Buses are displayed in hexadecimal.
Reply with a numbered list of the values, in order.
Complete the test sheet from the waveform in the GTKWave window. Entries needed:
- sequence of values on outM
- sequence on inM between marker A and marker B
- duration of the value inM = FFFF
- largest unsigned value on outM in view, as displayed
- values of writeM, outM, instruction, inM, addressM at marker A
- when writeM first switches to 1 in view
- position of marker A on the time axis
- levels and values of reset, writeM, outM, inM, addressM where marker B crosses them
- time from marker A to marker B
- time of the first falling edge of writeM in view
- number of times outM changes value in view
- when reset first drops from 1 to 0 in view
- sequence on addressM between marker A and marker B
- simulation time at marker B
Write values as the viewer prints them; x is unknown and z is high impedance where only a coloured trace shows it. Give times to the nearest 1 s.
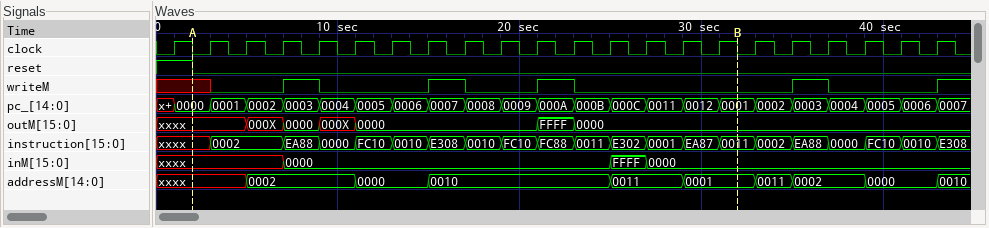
1. xxxx, 000X, 0000, 000X, 0000, FFFF, 0000
2. xxxx, 0000, FFFF, 0000
3. 2 s
4. FFFF
5. writeM=x, outM=xxxx, instruction=xxxx, inM=xxxx, addressM=xxxx
6. 7 s
7. 2 s
8. reset=0, writeM=0, outM=0000, inM=0000, addressM=0001
9. 30 s
10. 9 s
11. 6
12. 2 s
13. xxxx, 0002, 0000, 0010, 0011, 0001
14. 32 s
